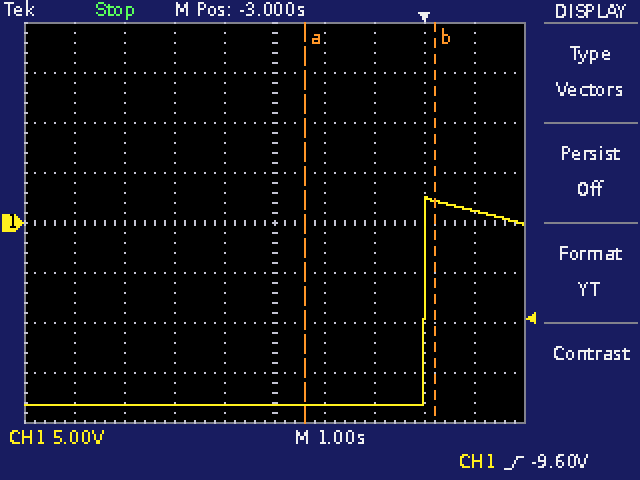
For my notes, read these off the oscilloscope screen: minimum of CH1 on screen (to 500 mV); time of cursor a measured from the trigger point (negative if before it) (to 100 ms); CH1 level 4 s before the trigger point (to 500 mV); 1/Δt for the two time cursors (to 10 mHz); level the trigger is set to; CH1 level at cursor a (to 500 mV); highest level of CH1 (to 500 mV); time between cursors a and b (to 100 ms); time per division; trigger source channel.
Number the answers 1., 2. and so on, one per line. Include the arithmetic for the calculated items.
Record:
1. -18.0 V
2. -2.4 s
3. -18.0 V
4. 1 / 2.6 s ≈ 380 mHz
5. -9.60 V
6. -18.0 V
7. 2.5 V
8. 2.6 s
9. 1 s
10. CH1
